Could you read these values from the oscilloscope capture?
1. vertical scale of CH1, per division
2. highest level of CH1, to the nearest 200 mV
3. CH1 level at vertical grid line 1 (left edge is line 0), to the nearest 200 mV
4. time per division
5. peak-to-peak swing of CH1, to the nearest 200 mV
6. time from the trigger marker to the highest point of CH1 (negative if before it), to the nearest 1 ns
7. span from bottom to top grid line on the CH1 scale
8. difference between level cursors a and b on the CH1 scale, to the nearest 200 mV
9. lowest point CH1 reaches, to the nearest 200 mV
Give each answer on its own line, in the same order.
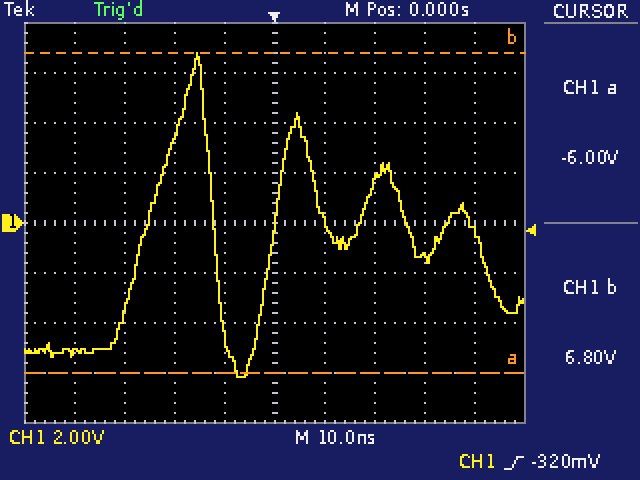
2 V
6.8 V
-5.2 V
10 ns
13.0 V
-15 ns
16 V
12.8 V
-6.2 V
